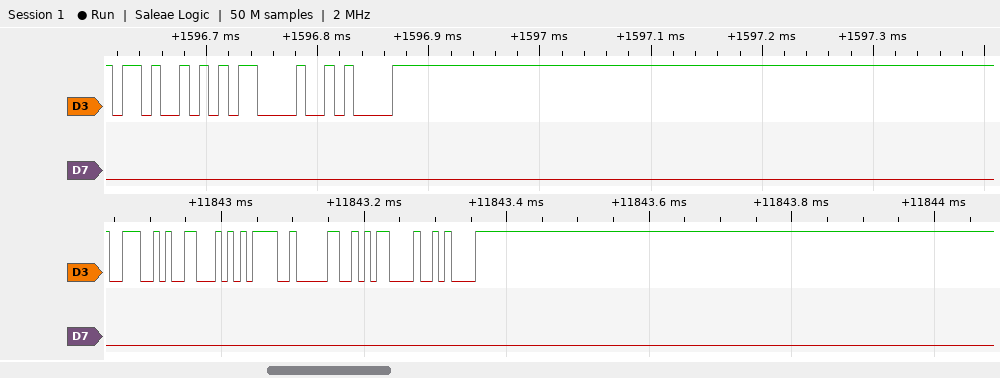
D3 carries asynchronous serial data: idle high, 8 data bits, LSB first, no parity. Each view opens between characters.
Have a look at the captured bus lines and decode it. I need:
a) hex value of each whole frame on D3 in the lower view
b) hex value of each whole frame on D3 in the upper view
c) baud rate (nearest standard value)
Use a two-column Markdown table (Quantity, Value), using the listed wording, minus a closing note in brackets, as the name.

| Quantity | Value |
|---|---|
| hex value of each whole frame on D3 in the lower view | 4E, 46, 3D, 30, 0D, 0A |
| hex value of each whole frame on D3 in the upper view | 4B, 0D, 0A |
| baud rate | 115200 baud |
